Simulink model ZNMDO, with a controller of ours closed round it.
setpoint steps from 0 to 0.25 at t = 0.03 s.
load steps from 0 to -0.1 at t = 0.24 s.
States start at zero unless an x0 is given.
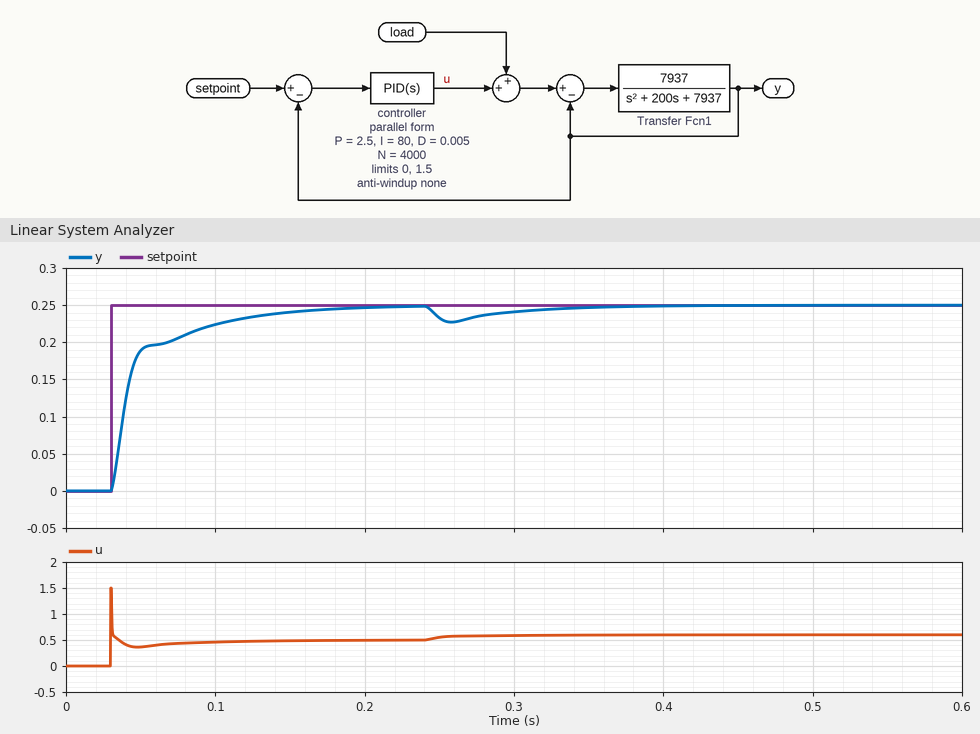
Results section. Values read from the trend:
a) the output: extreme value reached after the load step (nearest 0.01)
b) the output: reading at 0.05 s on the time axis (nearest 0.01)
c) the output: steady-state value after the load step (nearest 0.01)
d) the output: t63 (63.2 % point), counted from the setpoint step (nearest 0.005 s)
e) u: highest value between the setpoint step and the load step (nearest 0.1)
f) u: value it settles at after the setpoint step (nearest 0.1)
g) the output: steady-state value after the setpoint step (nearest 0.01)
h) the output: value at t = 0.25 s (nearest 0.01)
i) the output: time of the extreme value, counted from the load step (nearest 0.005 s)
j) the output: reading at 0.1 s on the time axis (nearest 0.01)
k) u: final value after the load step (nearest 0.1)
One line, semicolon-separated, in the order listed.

0.23; 0.19; 0.25; 0.015 s; 1.5; 0.5; 0.25; 0.23; 0.020 s; 0.22; 0.6
